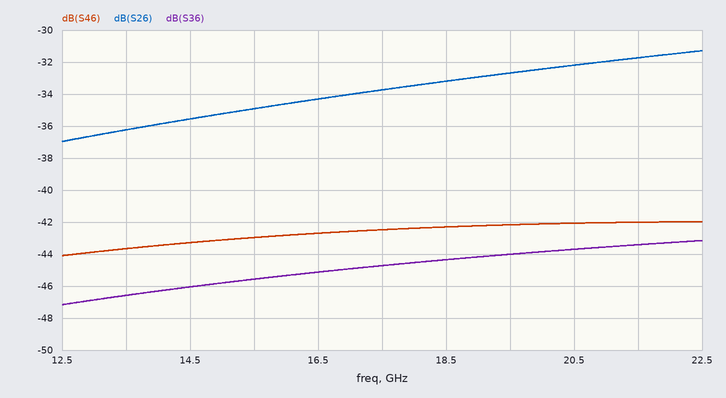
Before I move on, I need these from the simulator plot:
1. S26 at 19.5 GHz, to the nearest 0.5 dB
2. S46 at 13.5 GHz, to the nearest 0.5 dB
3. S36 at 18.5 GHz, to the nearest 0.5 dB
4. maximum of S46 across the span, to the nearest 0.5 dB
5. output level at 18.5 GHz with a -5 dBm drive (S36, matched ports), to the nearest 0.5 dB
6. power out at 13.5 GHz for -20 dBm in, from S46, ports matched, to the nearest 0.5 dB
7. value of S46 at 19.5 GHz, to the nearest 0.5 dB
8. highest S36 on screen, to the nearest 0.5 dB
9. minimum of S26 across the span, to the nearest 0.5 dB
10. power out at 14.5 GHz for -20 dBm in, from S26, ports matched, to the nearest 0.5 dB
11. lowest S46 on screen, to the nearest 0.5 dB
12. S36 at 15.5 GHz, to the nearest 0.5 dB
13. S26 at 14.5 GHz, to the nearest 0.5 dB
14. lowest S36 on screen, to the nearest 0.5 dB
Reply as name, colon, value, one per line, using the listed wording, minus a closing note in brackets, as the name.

S26 at 19.5 GHz, to the nearest 0.5 dB: -32.5 dB
S46 at 13.5 GHz, to the nearest 0.5 dB: -43.5 dB
S36 at 18.5 GHz, to the nearest 0.5 dB: -44.5 dB
maximum of S46 across the span, to the nearest 0.5 dB: -42.0 dB
output level at 18.5 GHz with a -5 dBm drive (S36, matched ports), to the nearest 0.5 dB: -49.5 dBm
power out at 13.5 GHz for -20 dBm in, from S46, ports matched, to the nearest 0.5 dB: -63.5 dBm
value of S46 at 19.5 GHz, to the nearest 0.5 dB: -42.0 dB
highest S36 on screen, to the nearest 0.5 dB: -43.0 dB
minimum of S26 across the span, to the nearest 0.5 dB: -37.0 dB
power out at 14.5 GHz for -20 dBm in, from S26, ports matched, to the nearest 0.5 dB: -55.5 dBm
lowest S46 on screen, to the nearest 0.5 dB: -44.0 dB
S36 at 15.5 GHz, to the nearest 0.5 dB: -45.5 dB
S26 at 14.5 GHz, to the nearest 0.5 dB: -35.5 dB
lowest S36 on screen, to the nearest 0.5 dB: -47.0 dB
